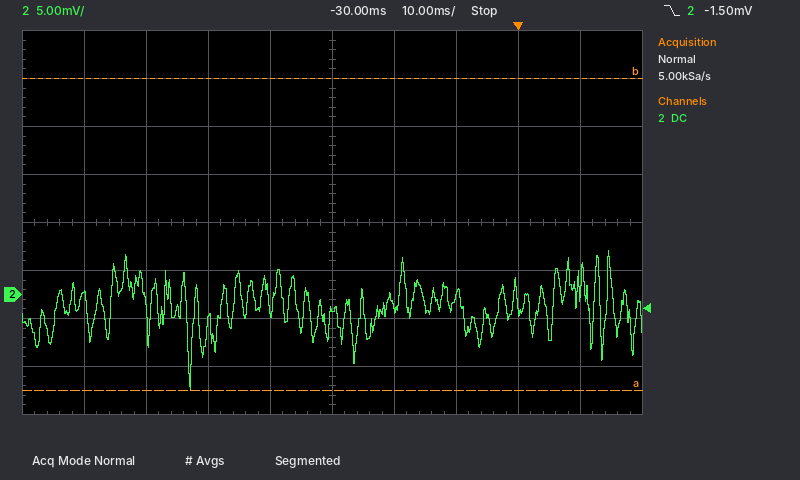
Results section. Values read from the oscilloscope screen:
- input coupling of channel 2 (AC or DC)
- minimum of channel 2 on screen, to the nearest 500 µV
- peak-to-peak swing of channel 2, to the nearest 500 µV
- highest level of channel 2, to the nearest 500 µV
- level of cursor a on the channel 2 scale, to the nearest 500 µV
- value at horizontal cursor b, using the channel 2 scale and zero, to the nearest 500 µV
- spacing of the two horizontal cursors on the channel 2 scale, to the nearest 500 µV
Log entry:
DC
-10.0 mV
14.5 mV
4.5 mV
-10.0 mV
22.5 mV
32.5 mV
